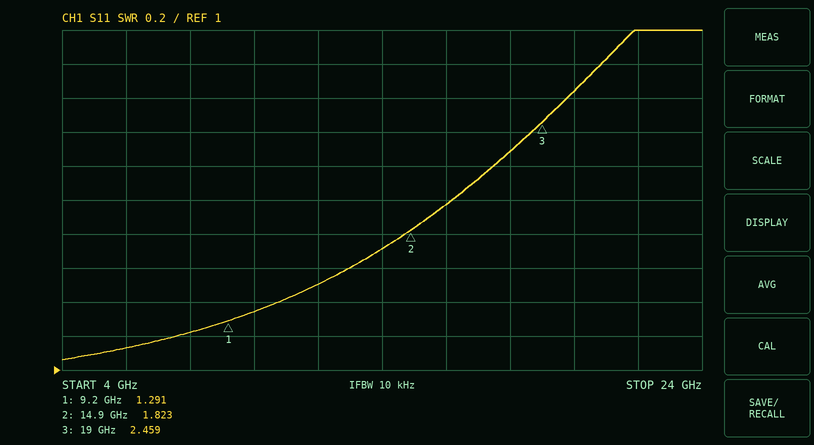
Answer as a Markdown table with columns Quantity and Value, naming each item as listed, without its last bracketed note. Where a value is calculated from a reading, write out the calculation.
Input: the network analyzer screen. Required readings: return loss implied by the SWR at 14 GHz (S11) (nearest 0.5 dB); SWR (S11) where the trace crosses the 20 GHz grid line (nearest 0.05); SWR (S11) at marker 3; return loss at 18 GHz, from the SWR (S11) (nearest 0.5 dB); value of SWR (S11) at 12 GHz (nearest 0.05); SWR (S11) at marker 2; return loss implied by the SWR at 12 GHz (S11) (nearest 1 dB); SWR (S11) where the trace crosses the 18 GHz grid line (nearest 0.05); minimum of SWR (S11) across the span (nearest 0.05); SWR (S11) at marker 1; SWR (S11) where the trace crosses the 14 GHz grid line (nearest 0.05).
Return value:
| Quantity | Value |
|---|---|
| return loss implied by the SWR at 14 GHz (S11) | −20 log10((1.7 − 1)/(1.7 + 1)) ≈ 11.7 dB, so 11.5 dB to the nearest 0.5 dB |
| SWR (S11) where the trace crosses the 20 GHz grid line | 2.65 |
| SWR (S11) at marker 3 | 2.459 |
| return loss at 18 GHz, from the SWR (S11) | −20 log10((2.3 − 1)/(2.3 + 1)) ≈ 8.09 dB, so 8.0 dB to the nearest 0.5 dB |
| value of SWR (S11) at 12 GHz | 1.50 |
| SWR (S11) at marker 2 | 1.823 |
| return loss implied by the SWR at 12 GHz (S11) | −20 log10((1.5 − 1)/(1.5 + 1)) ≈ 14 dB |
| SWR (S11) where the trace crosses the 18 GHz grid line | 2.30 |
| minimum of SWR (S11) across the span | 1.05 |
| SWR (S11) at marker 1 | 1.291 |
| SWR (S11) where the trace crosses the 14 GHz grid line | 1.70 |
